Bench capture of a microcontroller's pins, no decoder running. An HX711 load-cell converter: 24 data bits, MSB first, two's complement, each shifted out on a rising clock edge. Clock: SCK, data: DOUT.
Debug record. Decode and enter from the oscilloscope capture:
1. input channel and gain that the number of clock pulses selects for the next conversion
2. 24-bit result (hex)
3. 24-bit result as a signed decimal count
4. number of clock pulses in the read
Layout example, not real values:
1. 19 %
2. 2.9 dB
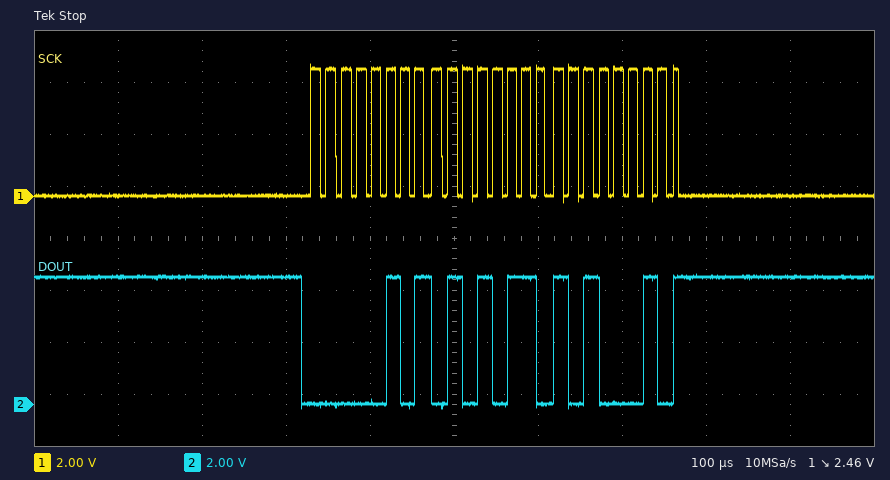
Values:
1. channel A, gain 128
2. 0x0556A2
3. 349858
4. 25
